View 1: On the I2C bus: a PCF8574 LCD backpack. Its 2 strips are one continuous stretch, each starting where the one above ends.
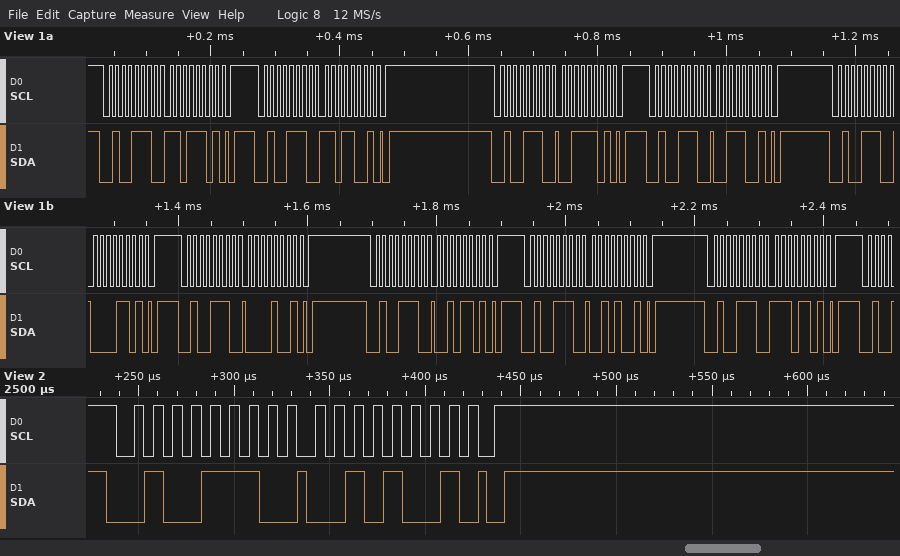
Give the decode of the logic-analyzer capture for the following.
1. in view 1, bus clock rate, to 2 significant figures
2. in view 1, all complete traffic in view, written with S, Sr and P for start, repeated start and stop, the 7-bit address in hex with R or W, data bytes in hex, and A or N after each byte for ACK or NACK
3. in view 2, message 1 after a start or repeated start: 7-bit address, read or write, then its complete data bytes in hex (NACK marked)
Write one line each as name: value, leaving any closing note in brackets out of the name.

in view 1, bus clock rate, to 2 significant figures: 100 kHz
in view 1, all complete traffic in view, written with S, Sr and P for start, repeated start and stop, the 7-bit address in hex with R or W, data bytes in hex, and A or N after each byte for ACK or NACK: S 27W A DD A P S 27W A D9 A P S 27W A 3D A P S 27W A 39 A P S 27W A 0D A P S 27W A 09 A P S 27W A 2D A P S 27W A 29 A P S 27W A ED A P
in view 2, message 1 after a start or repeated start: 7-bit address, read or write, then its complete data bytes in hex: 0x27 write: 29
